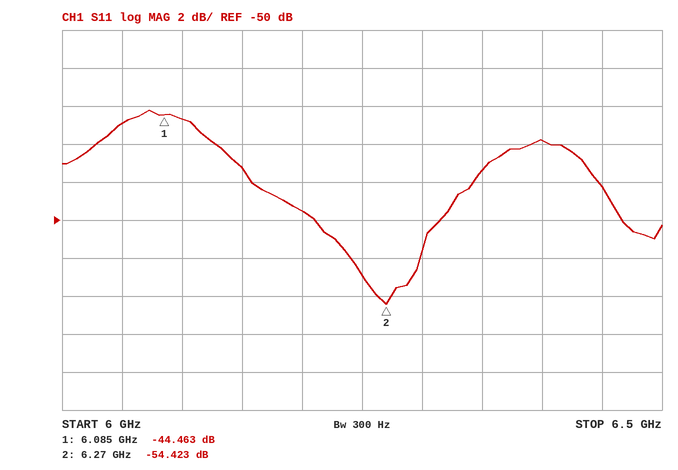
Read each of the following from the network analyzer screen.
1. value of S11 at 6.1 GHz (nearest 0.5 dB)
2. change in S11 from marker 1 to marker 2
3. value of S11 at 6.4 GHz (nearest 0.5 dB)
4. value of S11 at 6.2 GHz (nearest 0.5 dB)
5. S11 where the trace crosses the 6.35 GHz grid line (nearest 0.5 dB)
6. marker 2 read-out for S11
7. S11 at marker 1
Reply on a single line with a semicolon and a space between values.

-44.5 dB; -9.960 dB; -46.0 dB; -49.5 dB; -47.5 dB; -54.423 dB; -44.463 dB
